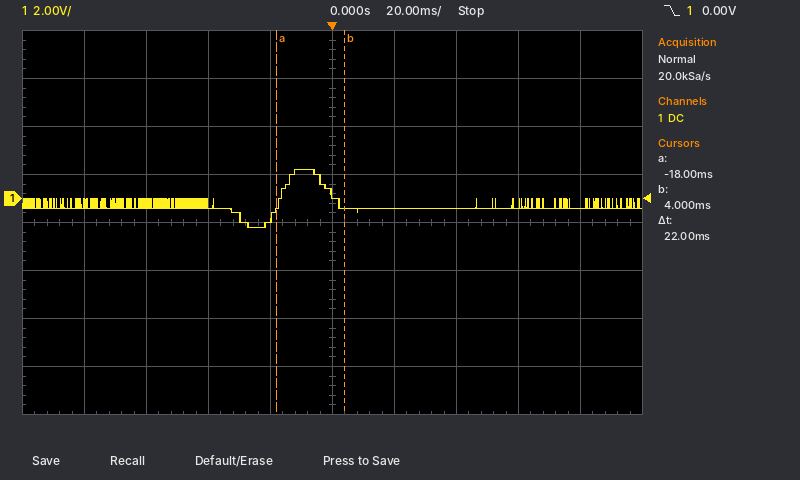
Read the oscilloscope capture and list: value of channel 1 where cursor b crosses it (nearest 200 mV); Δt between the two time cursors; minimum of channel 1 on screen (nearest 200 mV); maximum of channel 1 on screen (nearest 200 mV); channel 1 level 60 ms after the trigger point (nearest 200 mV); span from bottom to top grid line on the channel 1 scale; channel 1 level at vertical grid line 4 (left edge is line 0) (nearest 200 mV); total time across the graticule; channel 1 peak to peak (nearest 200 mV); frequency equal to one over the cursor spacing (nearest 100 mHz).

-400 mV
22 ms
-1.2 V
1.2 V
-200 mV
16 V
-800 mV
200 ms
2.4 V
45.5 Hz
